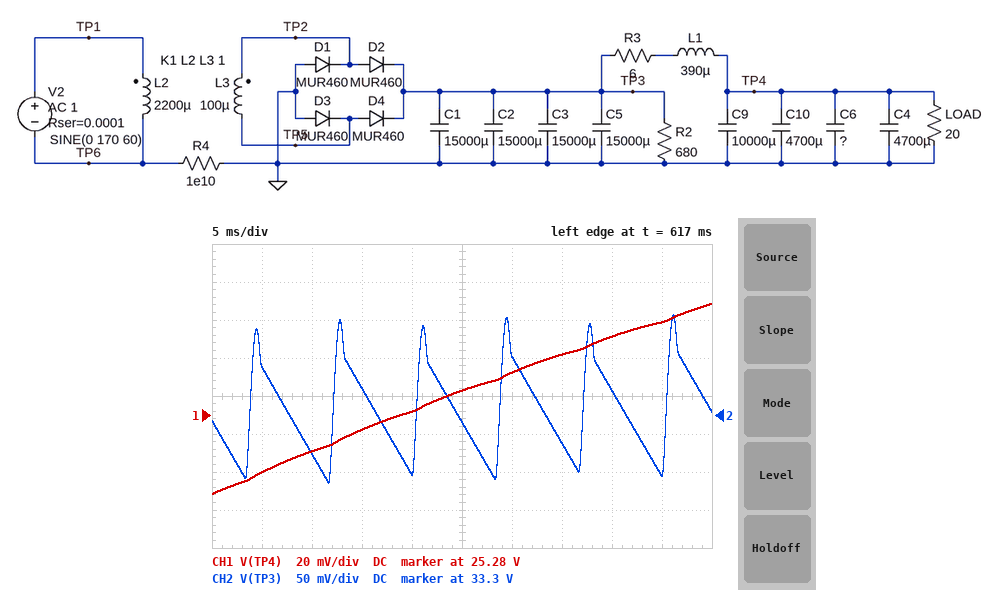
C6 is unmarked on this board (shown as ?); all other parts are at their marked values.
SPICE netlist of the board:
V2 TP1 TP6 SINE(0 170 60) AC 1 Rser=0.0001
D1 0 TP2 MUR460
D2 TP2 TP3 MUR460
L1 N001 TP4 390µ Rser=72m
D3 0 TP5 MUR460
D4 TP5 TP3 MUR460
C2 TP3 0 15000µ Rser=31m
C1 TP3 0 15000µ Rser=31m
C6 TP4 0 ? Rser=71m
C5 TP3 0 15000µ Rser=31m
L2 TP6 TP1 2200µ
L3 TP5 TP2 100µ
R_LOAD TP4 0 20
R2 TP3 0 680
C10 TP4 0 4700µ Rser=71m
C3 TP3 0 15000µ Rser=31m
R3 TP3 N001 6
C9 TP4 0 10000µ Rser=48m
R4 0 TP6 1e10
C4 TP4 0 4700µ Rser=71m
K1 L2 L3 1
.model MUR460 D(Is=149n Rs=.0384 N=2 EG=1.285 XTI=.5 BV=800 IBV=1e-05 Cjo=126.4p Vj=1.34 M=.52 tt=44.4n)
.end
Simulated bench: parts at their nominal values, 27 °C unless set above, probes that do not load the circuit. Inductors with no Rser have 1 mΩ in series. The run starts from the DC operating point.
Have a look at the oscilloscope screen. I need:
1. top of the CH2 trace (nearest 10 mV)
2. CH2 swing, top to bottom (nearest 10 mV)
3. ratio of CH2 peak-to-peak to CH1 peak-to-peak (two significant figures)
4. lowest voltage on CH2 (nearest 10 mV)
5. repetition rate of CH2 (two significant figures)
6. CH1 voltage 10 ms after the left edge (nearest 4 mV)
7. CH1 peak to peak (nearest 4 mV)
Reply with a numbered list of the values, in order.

1. 33.43 V
2. 220 mV
3. 2.2
4. 33.21 V
5. 120 Hz
6. 25.260 V
7. 100 mV
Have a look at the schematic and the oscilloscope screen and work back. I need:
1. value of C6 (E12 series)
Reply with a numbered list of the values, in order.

1. 8.2 mF
